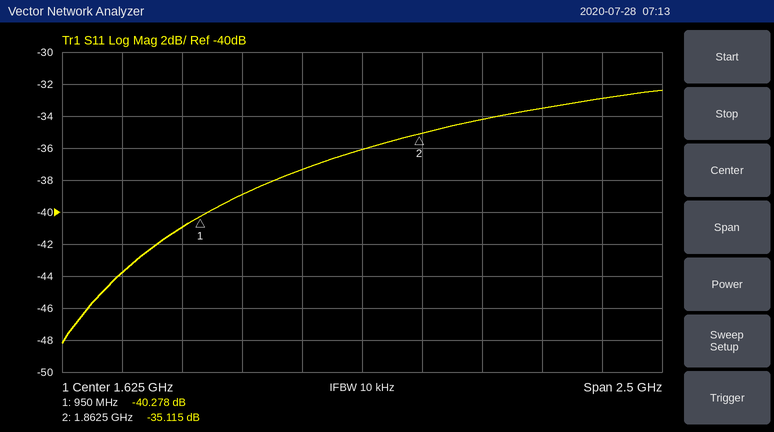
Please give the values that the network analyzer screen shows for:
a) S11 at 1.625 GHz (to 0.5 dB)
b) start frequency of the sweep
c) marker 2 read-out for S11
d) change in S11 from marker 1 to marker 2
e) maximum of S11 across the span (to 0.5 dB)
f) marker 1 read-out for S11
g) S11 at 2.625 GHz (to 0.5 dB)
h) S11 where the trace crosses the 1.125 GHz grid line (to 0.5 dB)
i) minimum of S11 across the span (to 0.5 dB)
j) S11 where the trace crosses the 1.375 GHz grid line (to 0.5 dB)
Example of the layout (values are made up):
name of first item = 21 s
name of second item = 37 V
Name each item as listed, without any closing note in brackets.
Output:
S11 at 1.625 GHz = -36.0 dB
start frequency of the sweep = 375 MHz
marker 2 read-out for S11 = -35.115 dB
change in S11 from marker 1 to marker 2 = 5.163 dB
maximum of S11 across the span = -32.5 dB
marker 1 read-out for S11 = -40.278 dB
S11 at 2.625 GHz = -33.0 dB
S11 where the trace crosses the 1.125 GHz grid line = -39.0 dB
minimum of S11 across the span = -48.0 dB
S11 where the trace crosses the 1.375 GHz grid line = -37.5 dB
